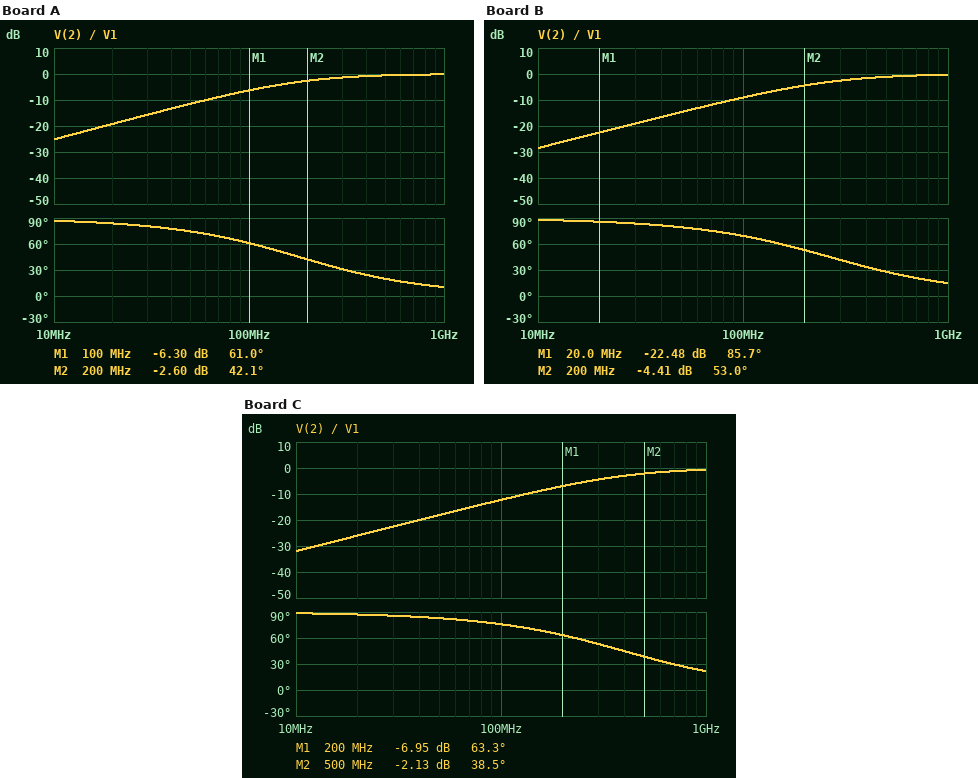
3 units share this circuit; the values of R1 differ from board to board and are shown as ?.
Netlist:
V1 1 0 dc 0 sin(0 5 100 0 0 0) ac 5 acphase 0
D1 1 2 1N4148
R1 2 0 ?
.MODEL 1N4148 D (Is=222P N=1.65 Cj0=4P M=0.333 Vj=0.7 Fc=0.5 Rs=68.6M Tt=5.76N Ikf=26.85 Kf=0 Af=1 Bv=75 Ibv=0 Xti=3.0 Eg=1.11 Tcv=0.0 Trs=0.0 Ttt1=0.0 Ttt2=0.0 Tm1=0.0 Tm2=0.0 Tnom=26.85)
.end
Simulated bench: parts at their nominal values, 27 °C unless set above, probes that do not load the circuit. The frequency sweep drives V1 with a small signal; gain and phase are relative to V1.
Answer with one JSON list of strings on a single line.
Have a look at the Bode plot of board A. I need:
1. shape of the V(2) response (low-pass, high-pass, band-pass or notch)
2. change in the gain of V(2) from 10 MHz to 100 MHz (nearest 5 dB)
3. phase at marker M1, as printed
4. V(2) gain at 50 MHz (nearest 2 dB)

["high-pass", "20 dB", "61.0 deg", "-12 dB"]
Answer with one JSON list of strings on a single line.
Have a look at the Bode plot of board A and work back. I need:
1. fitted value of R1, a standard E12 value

["220 Ω"]
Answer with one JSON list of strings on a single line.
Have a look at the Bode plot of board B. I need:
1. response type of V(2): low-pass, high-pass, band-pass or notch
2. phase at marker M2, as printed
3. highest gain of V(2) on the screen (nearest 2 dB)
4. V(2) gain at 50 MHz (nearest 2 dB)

["high-pass", "53.0 deg", "0 dB", "-14 dB"]
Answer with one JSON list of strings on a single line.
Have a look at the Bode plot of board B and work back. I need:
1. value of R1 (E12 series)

["150 Ω"]
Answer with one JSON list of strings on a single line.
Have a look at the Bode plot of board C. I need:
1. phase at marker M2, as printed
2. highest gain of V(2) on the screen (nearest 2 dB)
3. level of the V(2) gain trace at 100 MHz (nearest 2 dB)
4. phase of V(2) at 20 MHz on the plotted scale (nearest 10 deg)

["38.5 deg", "0 dB", "-12 dB", "90 deg"]
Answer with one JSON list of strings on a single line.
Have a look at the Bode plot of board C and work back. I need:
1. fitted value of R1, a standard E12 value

["100 Ω"]
